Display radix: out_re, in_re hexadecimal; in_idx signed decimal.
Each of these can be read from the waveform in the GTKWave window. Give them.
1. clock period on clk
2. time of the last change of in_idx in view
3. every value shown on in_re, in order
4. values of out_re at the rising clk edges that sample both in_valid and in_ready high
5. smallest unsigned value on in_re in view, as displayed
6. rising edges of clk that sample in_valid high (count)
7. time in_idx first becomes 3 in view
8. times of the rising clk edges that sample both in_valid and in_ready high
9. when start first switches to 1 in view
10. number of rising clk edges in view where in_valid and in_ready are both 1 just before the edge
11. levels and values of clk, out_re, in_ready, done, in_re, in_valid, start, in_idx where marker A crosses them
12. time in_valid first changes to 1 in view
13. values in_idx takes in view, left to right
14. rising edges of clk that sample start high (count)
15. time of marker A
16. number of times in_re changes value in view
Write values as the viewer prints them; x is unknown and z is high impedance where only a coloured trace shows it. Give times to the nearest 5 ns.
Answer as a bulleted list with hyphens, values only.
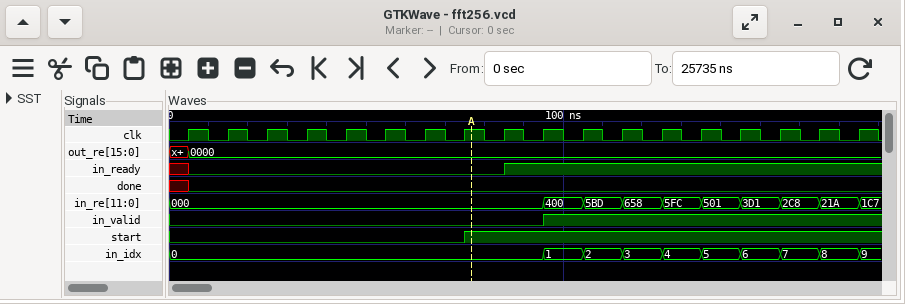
- 10 ns
- 175 ns
- 000, 400, 5BD, 658, 5FC, 501, 3D1, 2C8, 21A, 1C7
- 0000, 0000, 0000, 0000, 0000, 0000, 0000, 0000
- 000
- 8
- 115 ns
- 105 ns, 115 ns, 125 ns, 135 ns, 145 ns, 155 ns, 165 ns, 175 ns
- 75 ns
- 8
- clk=1, out_re=0000, in_ready=0, done=0, in_re=000, in_valid=0, start=1, in_idx=0
- 95 ns
- 0, 1, 2, 3, 4, 5, 6, 7, 8, 9
- 10
- 75 ns
- 9
